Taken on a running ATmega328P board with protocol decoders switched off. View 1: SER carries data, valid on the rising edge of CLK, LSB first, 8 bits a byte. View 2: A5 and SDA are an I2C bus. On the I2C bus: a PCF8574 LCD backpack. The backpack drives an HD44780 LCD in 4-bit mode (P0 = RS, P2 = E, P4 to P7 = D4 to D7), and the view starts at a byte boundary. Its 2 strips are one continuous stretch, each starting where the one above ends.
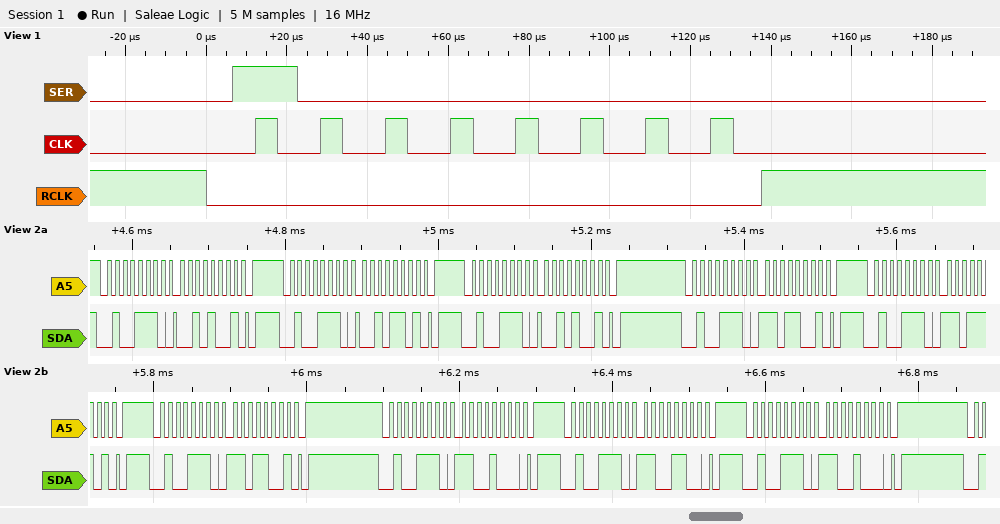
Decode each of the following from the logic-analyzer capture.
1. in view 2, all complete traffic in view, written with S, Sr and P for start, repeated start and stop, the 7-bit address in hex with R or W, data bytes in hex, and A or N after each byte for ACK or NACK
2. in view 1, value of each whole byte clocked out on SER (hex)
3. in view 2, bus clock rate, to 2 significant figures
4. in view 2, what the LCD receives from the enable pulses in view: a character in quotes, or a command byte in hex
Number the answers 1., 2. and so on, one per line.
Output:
1. S 27W A 29 A P S 27W A 2D A P S 27W A 29 A P S 27W A D9 A P S 27W A DD A P S 27W A D9 A P S 27W A C8 A P S 27W A CC A P S 27W A C8 A P
2. 01
3. 100 kHz
4. '-'
